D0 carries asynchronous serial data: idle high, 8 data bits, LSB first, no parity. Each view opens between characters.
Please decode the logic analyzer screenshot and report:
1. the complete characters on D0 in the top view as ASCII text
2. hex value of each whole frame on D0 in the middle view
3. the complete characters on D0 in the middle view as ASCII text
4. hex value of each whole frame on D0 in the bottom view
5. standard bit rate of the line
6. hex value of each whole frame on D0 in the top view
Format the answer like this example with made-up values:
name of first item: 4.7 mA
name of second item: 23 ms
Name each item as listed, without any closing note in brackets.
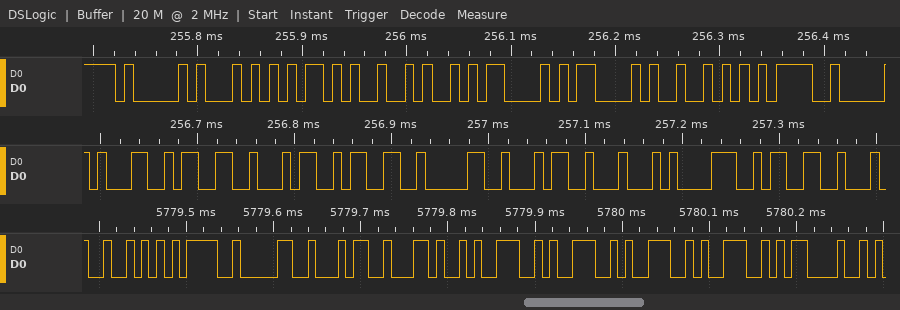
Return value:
the complete characters on D0 in the top view as ASCII text: "AT+JCCR="
hex value of each whole frame on D0 in the middle view: 31, 33, 34, 33, 30, 34, 44, 38, 33
the complete characters on D0 in the middle view as ASCII text: "134304D83"
hex value of each whole frame on D0 in the bottom view: 52, 3D, 30, 34, 2C, 39, 39, 39, 39, 0D
standard bit rate of the line: 115200 baud
hex value of each whole frame on D0 in the top view: 41, 54, 2B, 4A, 43, 43, 52, 3D
